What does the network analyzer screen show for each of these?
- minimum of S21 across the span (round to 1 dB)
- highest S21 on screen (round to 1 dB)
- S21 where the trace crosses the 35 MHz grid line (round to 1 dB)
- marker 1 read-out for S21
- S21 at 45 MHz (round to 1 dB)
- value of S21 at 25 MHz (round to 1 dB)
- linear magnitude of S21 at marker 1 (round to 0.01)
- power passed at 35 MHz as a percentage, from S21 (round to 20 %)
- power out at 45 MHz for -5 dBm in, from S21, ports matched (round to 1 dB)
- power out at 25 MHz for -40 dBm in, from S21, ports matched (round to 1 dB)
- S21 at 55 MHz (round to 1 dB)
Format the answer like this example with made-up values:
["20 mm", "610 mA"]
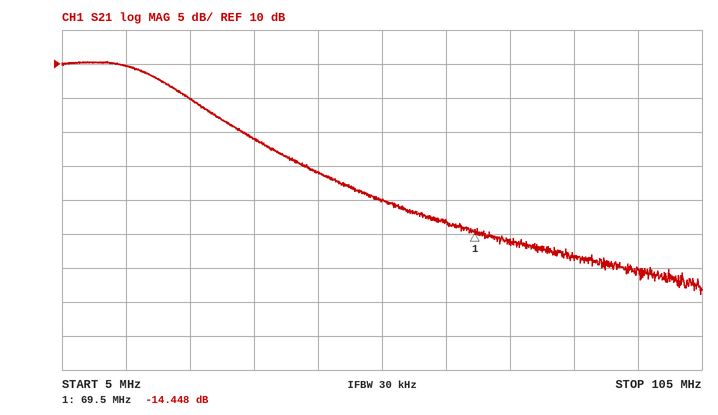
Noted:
["-24 dB", "10 dB", "-1 dB", "-14.448 dB", "-6 dB", "5 dB", "0.19", "80 %", "-11 dBm", "-35 dBm", "-10 dB"]
